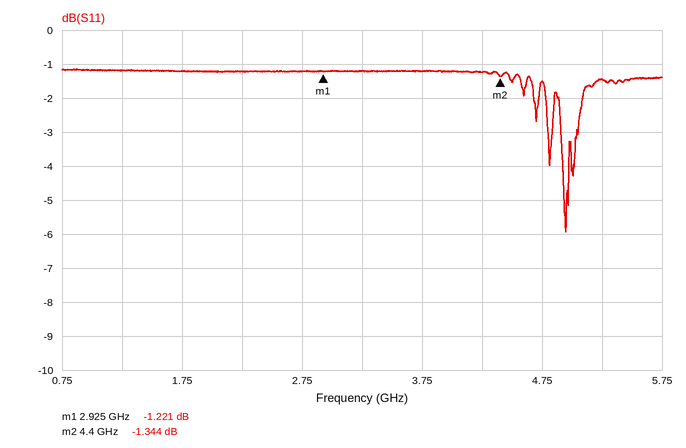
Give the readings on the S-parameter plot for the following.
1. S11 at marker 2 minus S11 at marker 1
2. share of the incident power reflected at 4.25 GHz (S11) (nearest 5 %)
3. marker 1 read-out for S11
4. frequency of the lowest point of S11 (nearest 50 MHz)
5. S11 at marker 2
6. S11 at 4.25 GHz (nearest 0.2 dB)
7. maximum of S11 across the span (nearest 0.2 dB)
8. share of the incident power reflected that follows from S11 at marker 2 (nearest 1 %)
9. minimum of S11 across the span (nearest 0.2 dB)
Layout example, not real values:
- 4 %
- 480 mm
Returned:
- -0.123 dB
- 75 %
- -1.221 dB
- 4.95 GHz
- -1.344 dB
- -1.2 dB
- -1.2 dB
- 73 %
- -6.0 dB
